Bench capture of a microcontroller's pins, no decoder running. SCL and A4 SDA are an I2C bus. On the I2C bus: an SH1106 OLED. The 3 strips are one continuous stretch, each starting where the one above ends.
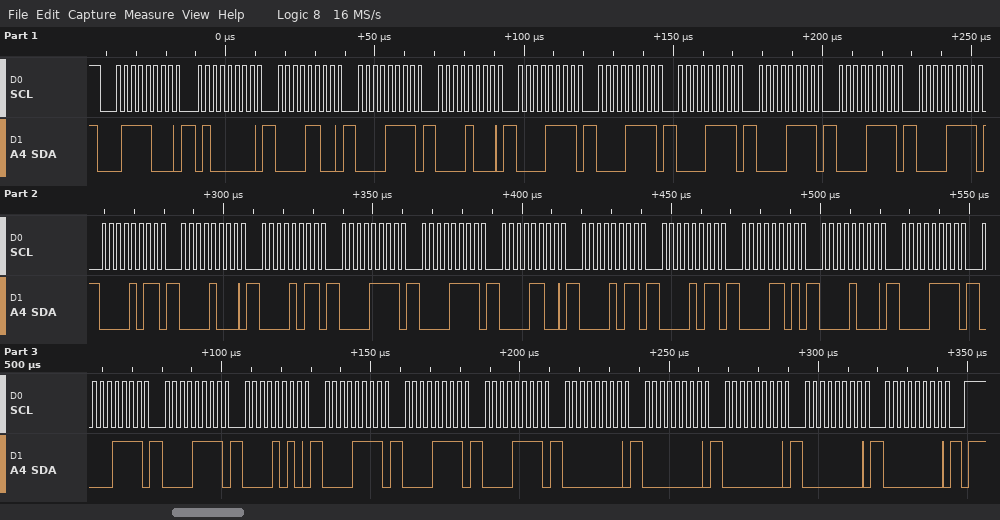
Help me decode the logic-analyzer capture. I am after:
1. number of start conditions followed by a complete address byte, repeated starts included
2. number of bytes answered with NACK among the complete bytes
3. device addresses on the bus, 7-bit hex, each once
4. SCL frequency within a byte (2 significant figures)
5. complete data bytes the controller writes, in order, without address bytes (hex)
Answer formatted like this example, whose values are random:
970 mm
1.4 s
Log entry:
1
0
0x3C
400 kHz
40 0C 0F 08 0F 0F 0F 0F 0F 0F 0B 08 0B 0F 0F 0C 0B 0B 0D 08 0F 0F 0F 0A 0F 0F 0F 00 00 00 00 00
